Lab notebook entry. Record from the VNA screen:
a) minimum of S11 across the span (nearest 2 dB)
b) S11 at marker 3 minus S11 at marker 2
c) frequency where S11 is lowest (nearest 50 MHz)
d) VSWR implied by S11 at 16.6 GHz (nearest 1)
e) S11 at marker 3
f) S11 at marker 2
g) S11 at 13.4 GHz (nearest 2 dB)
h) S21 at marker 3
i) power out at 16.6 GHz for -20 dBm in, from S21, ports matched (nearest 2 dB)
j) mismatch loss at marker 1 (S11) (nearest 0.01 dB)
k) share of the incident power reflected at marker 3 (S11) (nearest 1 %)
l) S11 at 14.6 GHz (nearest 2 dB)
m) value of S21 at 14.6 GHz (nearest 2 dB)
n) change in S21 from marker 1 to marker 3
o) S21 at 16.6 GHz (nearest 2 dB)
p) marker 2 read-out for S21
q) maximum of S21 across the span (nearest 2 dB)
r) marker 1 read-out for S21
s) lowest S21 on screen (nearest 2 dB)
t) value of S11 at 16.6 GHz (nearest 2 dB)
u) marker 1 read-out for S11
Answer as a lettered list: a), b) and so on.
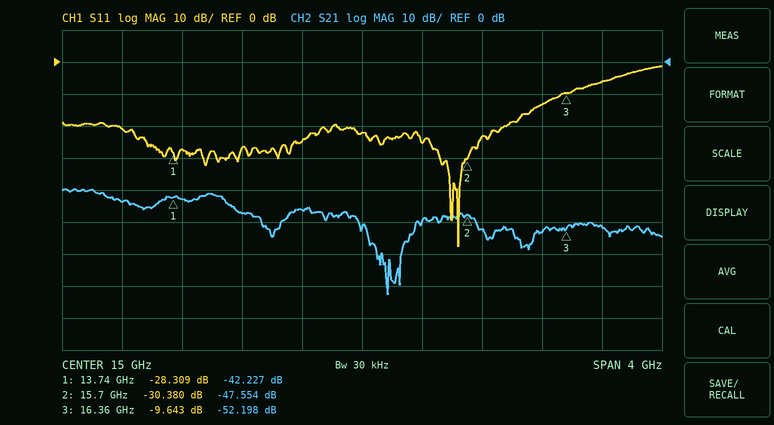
a) -58 dB
b) 20.737 dB
c) 15.65 GHz
d) 3
e) -9.643 dB
f) -30.380 dB
g) -20 dB
h) -52.198 dB
i) -72 dBm
j) 0.01 dB
k) 11 %
l) -24 dB
m) -46 dB
n) -9.971 dB
o) -52 dB
p) -47.554 dB
q) -40 dB
r) -42.227 dB
s) -72 dB
t) -6 dB
u) -28.309 dB
